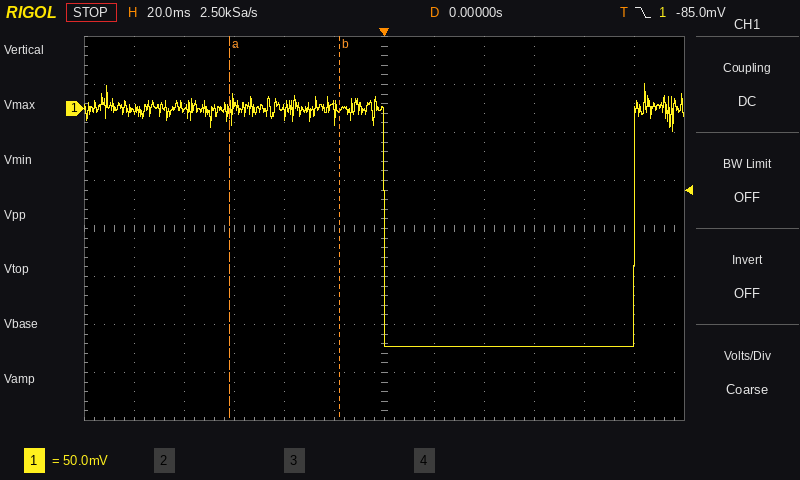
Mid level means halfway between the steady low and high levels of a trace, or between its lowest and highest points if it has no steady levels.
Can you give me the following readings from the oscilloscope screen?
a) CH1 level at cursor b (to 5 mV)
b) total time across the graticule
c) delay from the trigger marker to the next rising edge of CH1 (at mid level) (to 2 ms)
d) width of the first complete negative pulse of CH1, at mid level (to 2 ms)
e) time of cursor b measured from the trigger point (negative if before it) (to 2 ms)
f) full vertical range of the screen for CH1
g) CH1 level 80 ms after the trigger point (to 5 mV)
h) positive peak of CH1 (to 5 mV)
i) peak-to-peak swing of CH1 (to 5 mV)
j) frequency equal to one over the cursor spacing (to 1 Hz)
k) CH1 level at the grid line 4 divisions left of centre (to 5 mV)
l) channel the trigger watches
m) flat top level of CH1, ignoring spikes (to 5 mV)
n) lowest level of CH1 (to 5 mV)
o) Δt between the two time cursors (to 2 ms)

0 mV
240 ms
100 ms
100 ms
-18 ms
400 mV
-250 mV
25 mV
275 mV
23 Hz
0 mV
CH1
0 mV
-250 mV
44 ms
